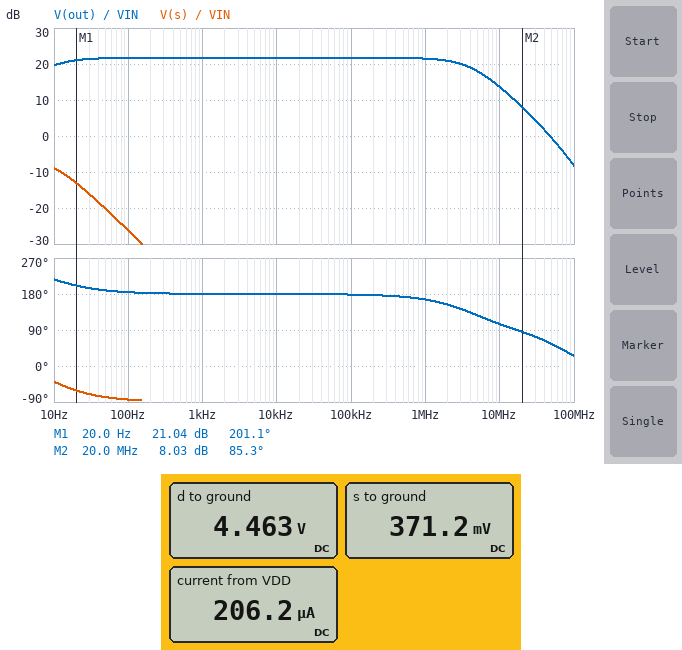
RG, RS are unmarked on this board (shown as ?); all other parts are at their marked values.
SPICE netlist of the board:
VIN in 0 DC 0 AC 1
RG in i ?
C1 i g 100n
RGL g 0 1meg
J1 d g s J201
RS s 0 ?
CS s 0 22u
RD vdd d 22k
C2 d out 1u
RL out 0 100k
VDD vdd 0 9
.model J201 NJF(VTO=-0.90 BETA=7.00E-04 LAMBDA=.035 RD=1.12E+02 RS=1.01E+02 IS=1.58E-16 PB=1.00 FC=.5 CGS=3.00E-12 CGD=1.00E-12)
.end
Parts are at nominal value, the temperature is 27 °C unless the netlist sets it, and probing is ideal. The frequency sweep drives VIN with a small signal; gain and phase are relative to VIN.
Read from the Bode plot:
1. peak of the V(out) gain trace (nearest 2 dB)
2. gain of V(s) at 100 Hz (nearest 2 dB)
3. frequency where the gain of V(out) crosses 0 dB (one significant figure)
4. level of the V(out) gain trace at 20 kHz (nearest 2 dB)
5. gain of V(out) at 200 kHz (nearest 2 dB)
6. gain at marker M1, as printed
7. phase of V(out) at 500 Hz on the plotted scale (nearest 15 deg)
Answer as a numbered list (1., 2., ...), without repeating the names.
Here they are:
1. 22 dB
2. -26 dB
3. 50 MHz
4. 22 dB
5. 22 dB
6. 21.04 dB
7. 180 deg
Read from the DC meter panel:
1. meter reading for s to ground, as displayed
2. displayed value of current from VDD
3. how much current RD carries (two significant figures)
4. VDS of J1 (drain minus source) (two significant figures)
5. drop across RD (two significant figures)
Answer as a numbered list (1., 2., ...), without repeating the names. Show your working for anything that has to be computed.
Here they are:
1. 371.2 mV
2. 206.2 µA
3. (9 V - 4.463 V) / 22 kΩ = 210 µA
4. 4.463 V - 371.2 mV = 4.1 V
5. 9 V - 4.463 V = 4.5 V
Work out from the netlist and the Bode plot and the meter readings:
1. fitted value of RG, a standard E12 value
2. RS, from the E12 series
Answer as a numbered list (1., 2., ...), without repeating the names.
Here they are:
1. 3.9 kΩ
2. 1.8 kΩ
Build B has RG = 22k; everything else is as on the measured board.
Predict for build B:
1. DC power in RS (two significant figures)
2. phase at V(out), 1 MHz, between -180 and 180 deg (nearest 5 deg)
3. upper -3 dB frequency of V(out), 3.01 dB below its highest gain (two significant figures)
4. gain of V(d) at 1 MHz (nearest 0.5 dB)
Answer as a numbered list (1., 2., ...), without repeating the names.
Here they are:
1. 77 µW
2. 130 deg
3. 890 kHz
4. 18.0 dB
